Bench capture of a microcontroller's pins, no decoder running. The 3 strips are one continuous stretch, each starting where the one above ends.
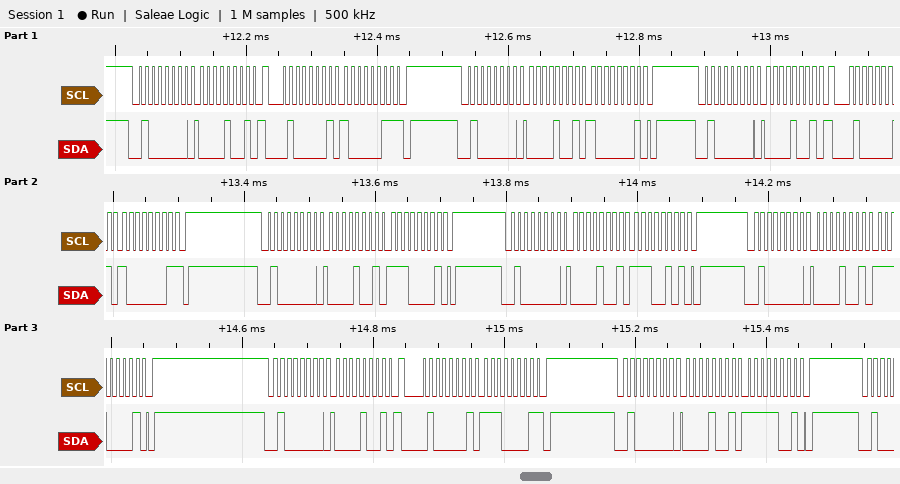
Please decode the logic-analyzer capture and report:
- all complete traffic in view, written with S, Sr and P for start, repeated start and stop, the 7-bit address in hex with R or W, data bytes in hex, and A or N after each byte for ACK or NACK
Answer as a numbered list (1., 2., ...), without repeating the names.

1. S 20W A 09 A Sr 20R A 83 N P S 20W A 09 A 81 A P S 20W A 09 A Sr 20R A 81 N P S 20W A 09 A E1 A P S 20W A 09 A E5 A P S 20W A 09 A E1 A P S 20W A 09 A Sr 20R A E1 N P S 20W A 09 A F9 A P
